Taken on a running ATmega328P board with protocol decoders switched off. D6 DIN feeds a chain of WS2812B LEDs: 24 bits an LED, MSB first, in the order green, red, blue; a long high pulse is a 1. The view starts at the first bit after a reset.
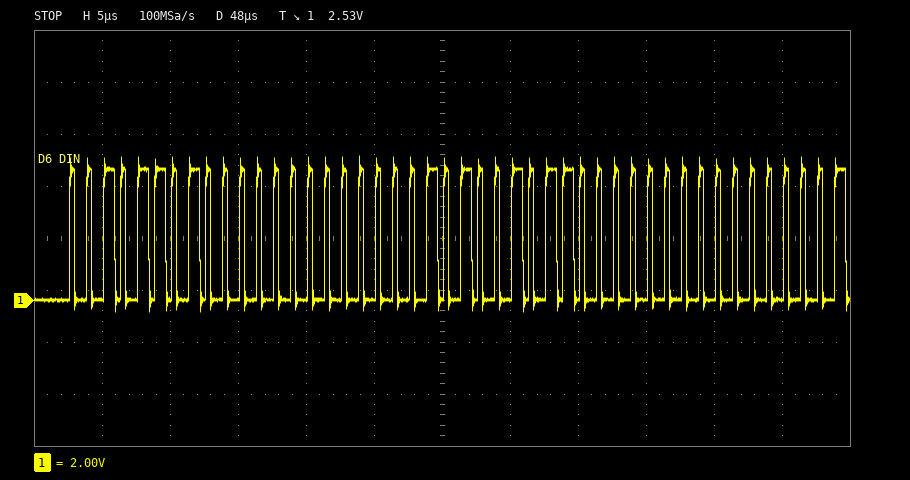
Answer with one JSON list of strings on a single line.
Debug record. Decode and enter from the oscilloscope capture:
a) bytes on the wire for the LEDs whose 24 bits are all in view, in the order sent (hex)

["2D 00 05"]
